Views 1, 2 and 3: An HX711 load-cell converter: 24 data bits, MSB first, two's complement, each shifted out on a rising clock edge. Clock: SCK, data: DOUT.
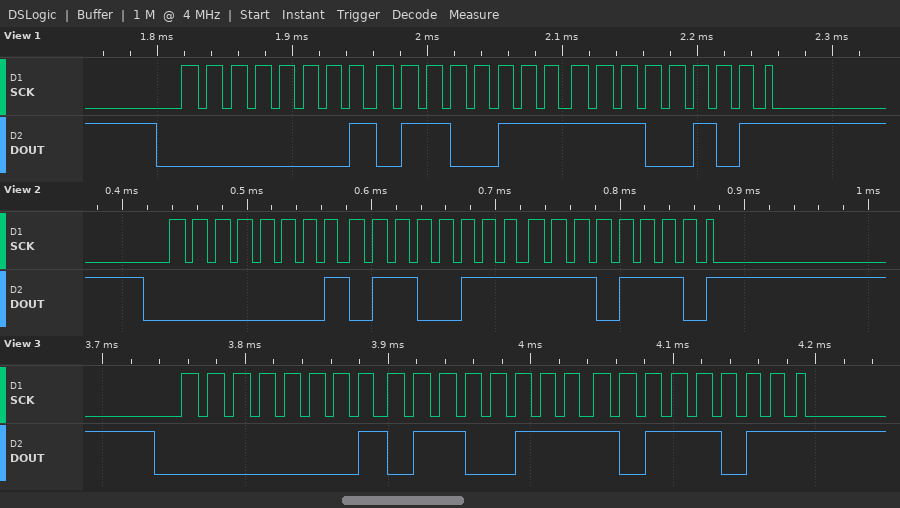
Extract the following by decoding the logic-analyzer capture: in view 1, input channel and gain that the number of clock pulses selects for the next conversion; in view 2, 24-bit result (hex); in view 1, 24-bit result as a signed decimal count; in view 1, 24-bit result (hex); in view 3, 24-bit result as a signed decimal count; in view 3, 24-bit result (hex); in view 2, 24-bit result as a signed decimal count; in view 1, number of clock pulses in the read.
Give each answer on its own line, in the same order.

channel A, gain 128
0x0167EE
92133
0x0167E5
92091
0x0167BB
92142
25
